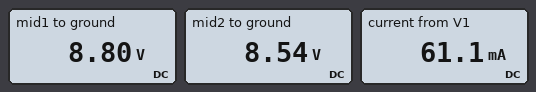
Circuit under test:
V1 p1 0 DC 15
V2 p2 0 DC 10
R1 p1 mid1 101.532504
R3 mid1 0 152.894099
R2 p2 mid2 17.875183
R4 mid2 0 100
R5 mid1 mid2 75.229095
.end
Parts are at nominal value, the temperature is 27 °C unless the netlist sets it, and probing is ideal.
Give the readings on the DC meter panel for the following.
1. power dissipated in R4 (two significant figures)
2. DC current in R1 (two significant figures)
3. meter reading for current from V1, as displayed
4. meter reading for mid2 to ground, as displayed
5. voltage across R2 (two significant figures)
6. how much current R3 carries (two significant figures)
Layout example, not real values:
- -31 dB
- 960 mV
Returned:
- 730 mW
- 61 mA
- 61.1 mA
- 8.54 V
- 1.5 V
- 58 mA
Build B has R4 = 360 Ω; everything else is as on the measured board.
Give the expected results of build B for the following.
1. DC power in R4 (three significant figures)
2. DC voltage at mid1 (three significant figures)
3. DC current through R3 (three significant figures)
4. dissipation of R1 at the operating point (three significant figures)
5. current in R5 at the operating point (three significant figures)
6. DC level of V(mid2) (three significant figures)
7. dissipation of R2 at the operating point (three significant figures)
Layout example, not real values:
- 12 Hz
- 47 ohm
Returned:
- 249 mW
- 9.22 V
- 60.3 mA
- 329 mW
- 3.35 mA
- 9.47 V
- 15.7 mW
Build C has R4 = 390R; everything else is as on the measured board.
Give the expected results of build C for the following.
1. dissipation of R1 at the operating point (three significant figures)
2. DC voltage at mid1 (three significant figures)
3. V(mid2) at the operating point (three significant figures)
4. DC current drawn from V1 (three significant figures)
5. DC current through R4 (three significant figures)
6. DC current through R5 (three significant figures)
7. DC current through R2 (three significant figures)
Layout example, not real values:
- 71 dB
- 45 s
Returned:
- 328 mW
- 9.23 V
- 9.50 V
- 56.8 mA
- 24.4 mA
- 3.57 mA
- 27.9 mA
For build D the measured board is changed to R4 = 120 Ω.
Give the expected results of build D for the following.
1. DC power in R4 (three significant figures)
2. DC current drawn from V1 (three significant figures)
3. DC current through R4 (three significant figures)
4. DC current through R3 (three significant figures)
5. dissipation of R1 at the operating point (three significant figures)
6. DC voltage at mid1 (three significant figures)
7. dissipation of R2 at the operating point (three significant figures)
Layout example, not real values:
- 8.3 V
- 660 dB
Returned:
- 636 mW
- 60.2 mA
- 72.8 mA
- 58.1 mA
- 368 mW
- 8.89 V
- 89.5 mW
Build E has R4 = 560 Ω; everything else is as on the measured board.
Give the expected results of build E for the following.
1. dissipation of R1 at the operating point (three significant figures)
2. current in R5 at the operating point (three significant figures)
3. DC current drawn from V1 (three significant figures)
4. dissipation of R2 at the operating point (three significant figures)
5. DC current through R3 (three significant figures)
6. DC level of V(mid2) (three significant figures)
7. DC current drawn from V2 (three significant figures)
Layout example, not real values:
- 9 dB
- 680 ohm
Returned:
- 322 mW
- 4.41 mA
- 56.3 mA
- 8.32 mW
- 60.7 mA
- 9.61 V
- 21.6 mA
